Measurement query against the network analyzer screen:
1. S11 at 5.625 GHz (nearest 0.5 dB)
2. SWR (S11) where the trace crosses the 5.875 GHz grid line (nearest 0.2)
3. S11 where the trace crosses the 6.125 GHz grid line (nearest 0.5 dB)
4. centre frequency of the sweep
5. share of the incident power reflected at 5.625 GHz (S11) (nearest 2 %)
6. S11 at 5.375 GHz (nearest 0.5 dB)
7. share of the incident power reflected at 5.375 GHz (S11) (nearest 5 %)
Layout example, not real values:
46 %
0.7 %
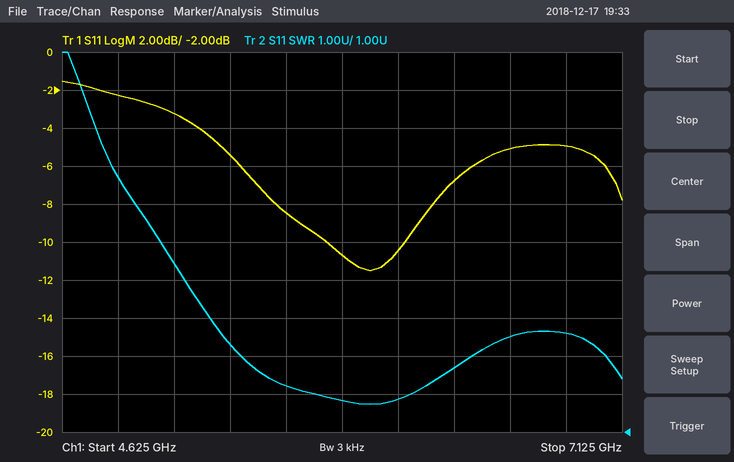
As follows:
-8.5 dB
1.8
-10.5 dB
5.875 GHz
14 %
-5.5 dB
30 %
